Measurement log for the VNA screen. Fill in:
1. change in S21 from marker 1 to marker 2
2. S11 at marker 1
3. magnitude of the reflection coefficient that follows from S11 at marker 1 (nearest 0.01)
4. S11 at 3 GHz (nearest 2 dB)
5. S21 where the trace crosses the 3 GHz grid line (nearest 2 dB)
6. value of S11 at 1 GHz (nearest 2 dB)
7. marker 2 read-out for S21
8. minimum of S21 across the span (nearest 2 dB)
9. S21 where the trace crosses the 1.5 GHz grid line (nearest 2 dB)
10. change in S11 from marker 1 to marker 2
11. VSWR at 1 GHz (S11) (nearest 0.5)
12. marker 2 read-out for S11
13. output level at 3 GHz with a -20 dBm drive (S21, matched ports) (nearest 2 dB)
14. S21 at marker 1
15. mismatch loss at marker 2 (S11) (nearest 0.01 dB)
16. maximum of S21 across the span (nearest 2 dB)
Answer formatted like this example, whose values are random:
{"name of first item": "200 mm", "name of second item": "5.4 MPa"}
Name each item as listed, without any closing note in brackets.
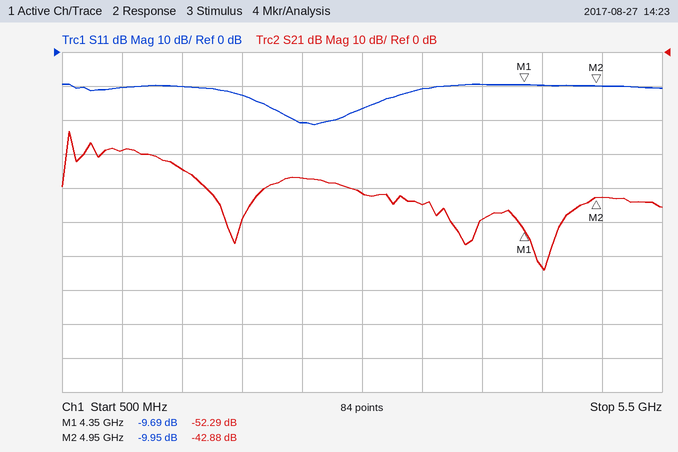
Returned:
{"change in S21 from marker 1 to marker 2": "9.41 dB", "S11 at marker 1": "-9.69 dB", "magnitude of the reflection coefficient that follows from S11 at marker 1": "0.33", "S11 at 3 GHz": "-16 dB", "S21 where the trace crosses the 3 GHz grid line": "-42 dB", "value of S11 at 1 GHz": "-10 dB", "marker 2 read-out for S21": "-42.88 dB", "minimum of S21 across the span": "-64 dB", "S21 where the trace crosses the 1.5 GHz grid line": "-34 dB", "change in S11 from marker 1 to marker 2": "-0.26 dB", "VSWR at 1 GHz (S11)": "2.0", "marker 2 read-out for S11": "-9.95 dB", "output level at 3 GHz with a -20 dBm drive (S21, matched ports)": "-62 dBm", "S21 at marker 1": "-52.29 dB", "mismatch loss at marker 2 (S11)": "0.46 dB", "maximum of S21 across the span": "-24 dB"}
